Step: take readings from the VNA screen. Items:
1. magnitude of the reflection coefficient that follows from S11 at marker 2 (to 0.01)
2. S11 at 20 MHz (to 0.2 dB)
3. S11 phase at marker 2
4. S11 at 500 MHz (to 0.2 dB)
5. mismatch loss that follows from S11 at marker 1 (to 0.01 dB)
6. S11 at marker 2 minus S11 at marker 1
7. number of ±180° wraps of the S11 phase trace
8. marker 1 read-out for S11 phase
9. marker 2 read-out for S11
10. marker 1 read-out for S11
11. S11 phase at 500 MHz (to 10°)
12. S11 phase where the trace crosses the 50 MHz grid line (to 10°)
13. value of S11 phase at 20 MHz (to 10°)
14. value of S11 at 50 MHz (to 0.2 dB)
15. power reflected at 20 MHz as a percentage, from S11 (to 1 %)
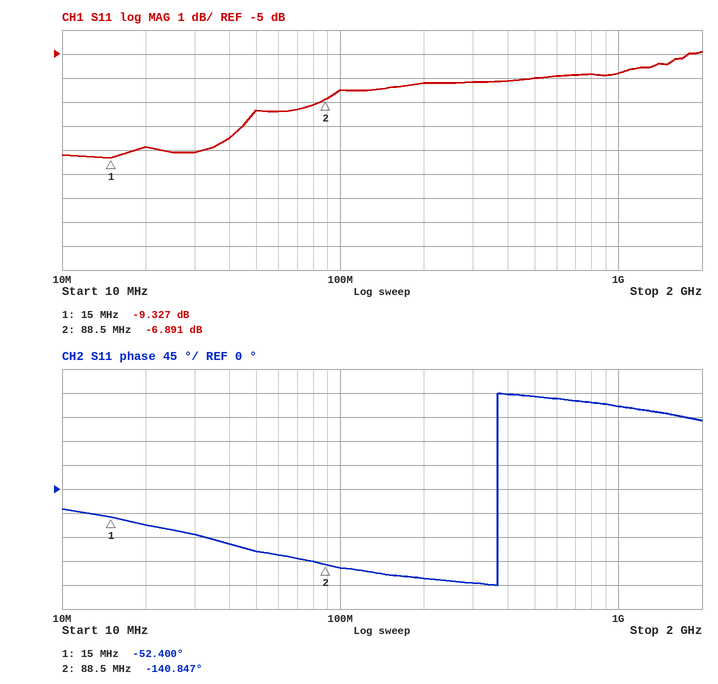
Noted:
0.45
-8.8 dB
-140.847°
-6.0 dB
0.54 dB
2.436 dB
1
-52.400°
-6.891 dB
-9.327 dB
170°
-120°
-70°
-7.4 dB
13 %
